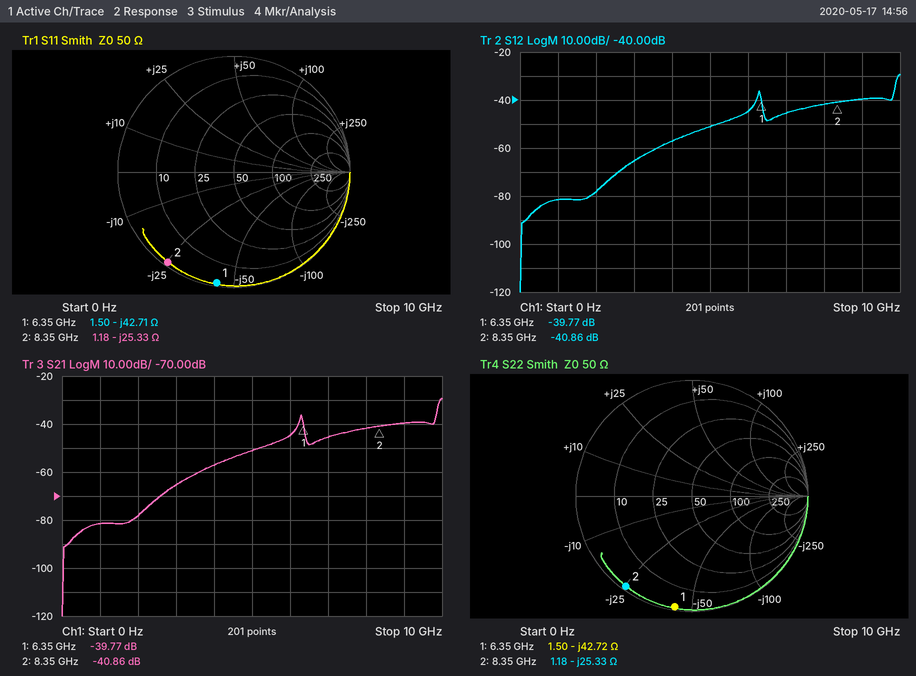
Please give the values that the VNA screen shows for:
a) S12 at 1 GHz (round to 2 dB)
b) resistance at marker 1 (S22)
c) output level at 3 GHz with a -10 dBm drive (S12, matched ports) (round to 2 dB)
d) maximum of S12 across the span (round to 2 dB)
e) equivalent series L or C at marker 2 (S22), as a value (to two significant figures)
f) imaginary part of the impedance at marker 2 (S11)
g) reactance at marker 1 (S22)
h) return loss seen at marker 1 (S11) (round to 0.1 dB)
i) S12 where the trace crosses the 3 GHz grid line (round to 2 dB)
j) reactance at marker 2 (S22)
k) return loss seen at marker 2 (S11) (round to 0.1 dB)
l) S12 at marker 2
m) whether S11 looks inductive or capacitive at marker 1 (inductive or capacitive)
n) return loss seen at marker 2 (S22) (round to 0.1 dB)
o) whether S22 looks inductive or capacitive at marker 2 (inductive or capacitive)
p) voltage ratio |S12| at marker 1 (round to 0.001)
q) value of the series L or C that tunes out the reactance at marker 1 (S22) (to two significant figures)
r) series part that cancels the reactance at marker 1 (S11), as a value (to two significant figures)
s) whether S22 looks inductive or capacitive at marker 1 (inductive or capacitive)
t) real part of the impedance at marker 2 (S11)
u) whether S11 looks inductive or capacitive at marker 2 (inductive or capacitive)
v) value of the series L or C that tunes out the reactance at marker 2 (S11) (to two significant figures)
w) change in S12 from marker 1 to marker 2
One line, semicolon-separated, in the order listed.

-82 dB; 1.50 Ω; -76 dBm; -30 dB; 750 fF; -25.33 Ω; -42.72 Ω; 0.3 dB; -66 dB; -25.33 Ω; 0.3 dB; -40.86 dB; capacitive; 0.3 dB; capacitive; 0.010; 1.1 nH; 1.1 nH; capacitive; 1.18 Ω; capacitive; 480 pH; -1.09 dB
